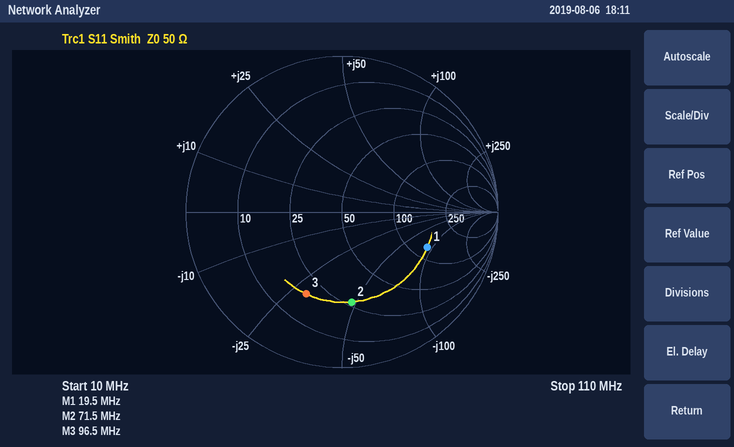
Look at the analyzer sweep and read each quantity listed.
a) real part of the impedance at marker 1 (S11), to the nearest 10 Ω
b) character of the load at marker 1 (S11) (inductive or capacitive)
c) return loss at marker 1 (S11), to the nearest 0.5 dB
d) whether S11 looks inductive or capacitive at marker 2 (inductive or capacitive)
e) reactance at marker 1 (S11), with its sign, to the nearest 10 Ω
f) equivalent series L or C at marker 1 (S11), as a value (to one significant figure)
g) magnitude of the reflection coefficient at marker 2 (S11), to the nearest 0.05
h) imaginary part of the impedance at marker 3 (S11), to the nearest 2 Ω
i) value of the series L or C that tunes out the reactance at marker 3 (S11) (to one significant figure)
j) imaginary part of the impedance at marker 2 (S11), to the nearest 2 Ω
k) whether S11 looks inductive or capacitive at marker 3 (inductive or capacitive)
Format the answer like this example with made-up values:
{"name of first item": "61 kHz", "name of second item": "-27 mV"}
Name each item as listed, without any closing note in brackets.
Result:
{"real part of the impedance at marker 1 (S11), to the nearest 10 Ω": "130 Ω", "character of the load at marker 1 (S11)": "capacitive", "return loss at marker 1 (S11), to the nearest 0.5 dB": "4.5 dB", "whether S11 looks inductive or capacitive at marker 2": "capacitive", "reactance at marker 1 (S11), with its sign, to the nearest 10 Ω": "-90 Ω", "equivalent series L or C at marker 1 (S11), as a value": "90 pF", "magnitude of the reflection coefficient at marker 2 (S11), to the nearest 0.05": "0.60", "imaginary part of the impedance at marker 3 (S11), to the nearest 2 Ω": "-30 Ω", "value of the series L or C that tunes out the reactance at marker 3 (S11)": "50 nH", "imaginary part of the impedance at marker 2 (S11), to the nearest 2 Ω": "-48 Ω", "whether S11 looks inductive or capacitive at marker 3": "capacitive"}
